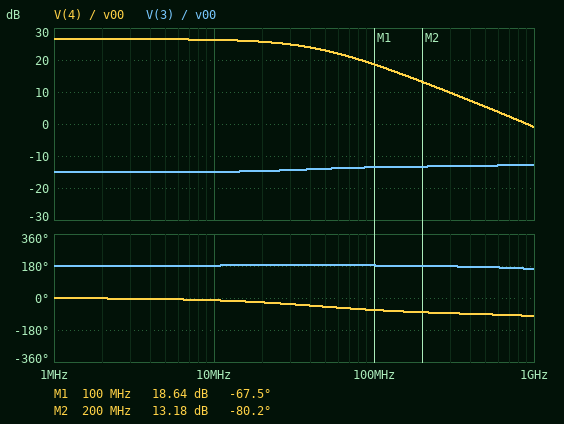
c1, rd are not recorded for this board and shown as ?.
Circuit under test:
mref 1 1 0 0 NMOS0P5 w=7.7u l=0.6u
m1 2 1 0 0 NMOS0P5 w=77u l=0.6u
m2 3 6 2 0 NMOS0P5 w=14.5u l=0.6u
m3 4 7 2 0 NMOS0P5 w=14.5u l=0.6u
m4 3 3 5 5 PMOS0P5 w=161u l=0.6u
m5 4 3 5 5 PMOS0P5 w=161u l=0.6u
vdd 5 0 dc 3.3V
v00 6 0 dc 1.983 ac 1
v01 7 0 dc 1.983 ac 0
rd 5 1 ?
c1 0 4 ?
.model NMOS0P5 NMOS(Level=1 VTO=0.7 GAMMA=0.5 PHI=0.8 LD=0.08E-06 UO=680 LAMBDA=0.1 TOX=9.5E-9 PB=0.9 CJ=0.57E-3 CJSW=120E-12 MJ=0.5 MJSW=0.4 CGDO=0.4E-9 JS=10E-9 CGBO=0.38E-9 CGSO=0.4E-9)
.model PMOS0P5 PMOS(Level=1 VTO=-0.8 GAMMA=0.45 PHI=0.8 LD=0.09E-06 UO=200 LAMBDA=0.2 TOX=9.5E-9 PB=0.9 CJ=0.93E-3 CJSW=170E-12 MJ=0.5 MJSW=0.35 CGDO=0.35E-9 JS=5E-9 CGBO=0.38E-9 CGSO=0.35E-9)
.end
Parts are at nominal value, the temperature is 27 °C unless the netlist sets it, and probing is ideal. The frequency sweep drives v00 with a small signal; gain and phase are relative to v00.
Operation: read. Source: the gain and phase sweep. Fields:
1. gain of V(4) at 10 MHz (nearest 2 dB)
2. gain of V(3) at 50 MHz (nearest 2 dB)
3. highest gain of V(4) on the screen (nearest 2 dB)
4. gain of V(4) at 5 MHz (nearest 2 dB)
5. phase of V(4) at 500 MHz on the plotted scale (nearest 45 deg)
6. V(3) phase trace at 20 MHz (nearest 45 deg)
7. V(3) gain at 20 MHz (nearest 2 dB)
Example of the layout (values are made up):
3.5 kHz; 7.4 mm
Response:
26 dB; -14 dB; 26 dB; 26 dB; -90 deg; 180 deg; -14 dB
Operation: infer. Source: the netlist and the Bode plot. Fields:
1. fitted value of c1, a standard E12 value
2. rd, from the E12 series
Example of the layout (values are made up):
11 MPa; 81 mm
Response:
470 fF; 18 kΩ
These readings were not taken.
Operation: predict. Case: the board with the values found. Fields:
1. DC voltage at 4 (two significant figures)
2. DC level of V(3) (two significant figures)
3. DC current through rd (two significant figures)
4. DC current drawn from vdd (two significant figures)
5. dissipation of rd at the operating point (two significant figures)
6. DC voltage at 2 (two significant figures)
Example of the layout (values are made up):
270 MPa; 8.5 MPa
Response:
2.3 V; 2.3 V; 130 µA; 1.4 mA; 310 µW; 740 mV
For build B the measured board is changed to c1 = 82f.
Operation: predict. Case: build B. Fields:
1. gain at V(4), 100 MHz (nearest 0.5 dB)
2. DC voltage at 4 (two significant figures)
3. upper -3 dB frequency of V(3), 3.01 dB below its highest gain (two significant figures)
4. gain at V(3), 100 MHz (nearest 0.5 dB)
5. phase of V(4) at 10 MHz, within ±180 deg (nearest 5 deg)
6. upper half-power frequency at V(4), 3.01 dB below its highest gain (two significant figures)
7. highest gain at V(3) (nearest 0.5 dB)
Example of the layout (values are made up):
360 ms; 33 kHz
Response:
24.5 dB; 2.3 V; 2.7 GHz; -16.0 dB; -5 deg; 130 MHz; -15.0 dB
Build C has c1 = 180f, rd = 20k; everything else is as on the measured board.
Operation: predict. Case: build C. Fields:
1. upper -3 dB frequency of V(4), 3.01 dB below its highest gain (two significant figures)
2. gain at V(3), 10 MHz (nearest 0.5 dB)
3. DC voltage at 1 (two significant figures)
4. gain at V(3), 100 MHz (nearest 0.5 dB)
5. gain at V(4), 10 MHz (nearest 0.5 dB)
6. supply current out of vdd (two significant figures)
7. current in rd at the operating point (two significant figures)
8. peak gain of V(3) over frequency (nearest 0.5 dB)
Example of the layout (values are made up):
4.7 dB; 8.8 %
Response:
79 MHz; -15.0 dB; 920 mV; -15.5 dB; 27.0 dB; 1.3 mA; 120 µA; -14.5 dB
